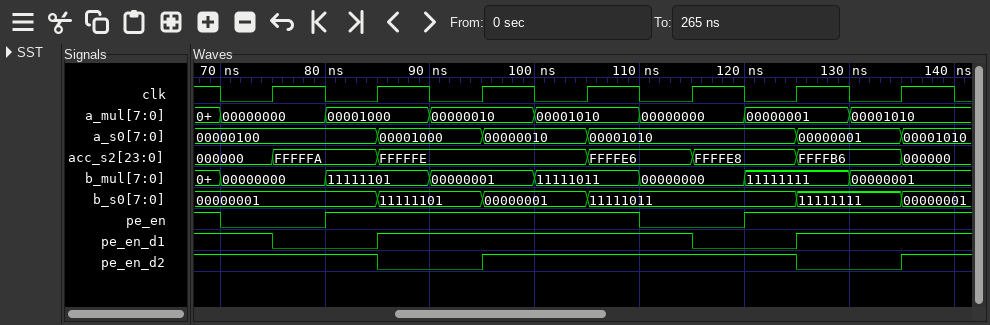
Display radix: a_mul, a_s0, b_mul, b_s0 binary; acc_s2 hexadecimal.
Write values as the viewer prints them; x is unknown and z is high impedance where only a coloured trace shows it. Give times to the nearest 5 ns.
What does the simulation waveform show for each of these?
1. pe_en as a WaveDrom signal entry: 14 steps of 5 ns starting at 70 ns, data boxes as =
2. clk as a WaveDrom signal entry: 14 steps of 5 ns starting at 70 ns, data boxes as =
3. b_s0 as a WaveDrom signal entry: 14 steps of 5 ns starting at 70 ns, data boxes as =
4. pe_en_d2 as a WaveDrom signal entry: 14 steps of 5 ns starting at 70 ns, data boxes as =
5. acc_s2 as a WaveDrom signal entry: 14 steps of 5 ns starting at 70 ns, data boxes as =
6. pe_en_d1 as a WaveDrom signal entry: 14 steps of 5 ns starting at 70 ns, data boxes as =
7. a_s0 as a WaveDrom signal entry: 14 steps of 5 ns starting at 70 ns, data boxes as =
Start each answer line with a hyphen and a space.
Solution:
- {name: 'pe_en', wave: '0.1.....0.1...'}
- {name: 'clk', wave: '01010101010101'}
- {name: 'b_s0', wave: '=..=.=.=...=.=', data: '00000001 11111101 00000001 11111011 11111111 00000001'}
- {name: 'pe_en_d2', wave: '1..0.1.....0.1'}
- {name: 'acc_s2', wave: '==.=...=.=.=.=', data: '000000 FFFFFA FFFFFE FFFFE6 FFFFE8 FFFFB6 000000'}
- {name: 'pe_en_d1', wave: '10.1.....0.1..'}
- {name: 'a_s0', wave: '=..=.=.=...=.=', data: '00000100 00001000 00000010 00001010 00000001 00001010'}
